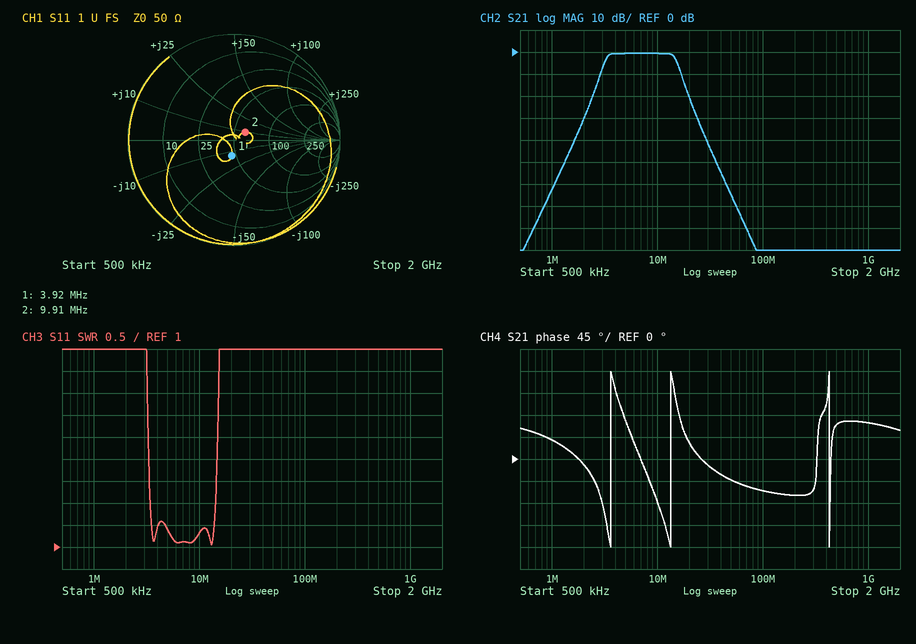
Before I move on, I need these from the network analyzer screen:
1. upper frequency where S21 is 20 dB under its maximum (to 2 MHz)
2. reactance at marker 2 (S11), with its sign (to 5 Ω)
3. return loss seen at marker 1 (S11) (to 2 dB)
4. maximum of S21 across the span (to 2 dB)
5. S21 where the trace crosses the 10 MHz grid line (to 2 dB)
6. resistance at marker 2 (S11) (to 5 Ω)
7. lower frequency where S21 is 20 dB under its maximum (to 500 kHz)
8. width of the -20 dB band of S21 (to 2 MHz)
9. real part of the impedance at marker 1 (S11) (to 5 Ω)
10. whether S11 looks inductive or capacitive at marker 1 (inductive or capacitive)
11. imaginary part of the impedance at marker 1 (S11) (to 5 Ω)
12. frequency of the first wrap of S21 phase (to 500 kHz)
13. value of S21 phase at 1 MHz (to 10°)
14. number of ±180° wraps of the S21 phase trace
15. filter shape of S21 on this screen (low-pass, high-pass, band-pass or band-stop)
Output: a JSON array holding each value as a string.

["20 MHz", "+10 Ω", "16 dB", "0 dB", "0 dB", "60 Ω", "2.5 MHz", "18 MHz", "45 Ω", "capacitive", "-15 Ω", "3.5 MHz", "40°", "3", "band-pass"]
